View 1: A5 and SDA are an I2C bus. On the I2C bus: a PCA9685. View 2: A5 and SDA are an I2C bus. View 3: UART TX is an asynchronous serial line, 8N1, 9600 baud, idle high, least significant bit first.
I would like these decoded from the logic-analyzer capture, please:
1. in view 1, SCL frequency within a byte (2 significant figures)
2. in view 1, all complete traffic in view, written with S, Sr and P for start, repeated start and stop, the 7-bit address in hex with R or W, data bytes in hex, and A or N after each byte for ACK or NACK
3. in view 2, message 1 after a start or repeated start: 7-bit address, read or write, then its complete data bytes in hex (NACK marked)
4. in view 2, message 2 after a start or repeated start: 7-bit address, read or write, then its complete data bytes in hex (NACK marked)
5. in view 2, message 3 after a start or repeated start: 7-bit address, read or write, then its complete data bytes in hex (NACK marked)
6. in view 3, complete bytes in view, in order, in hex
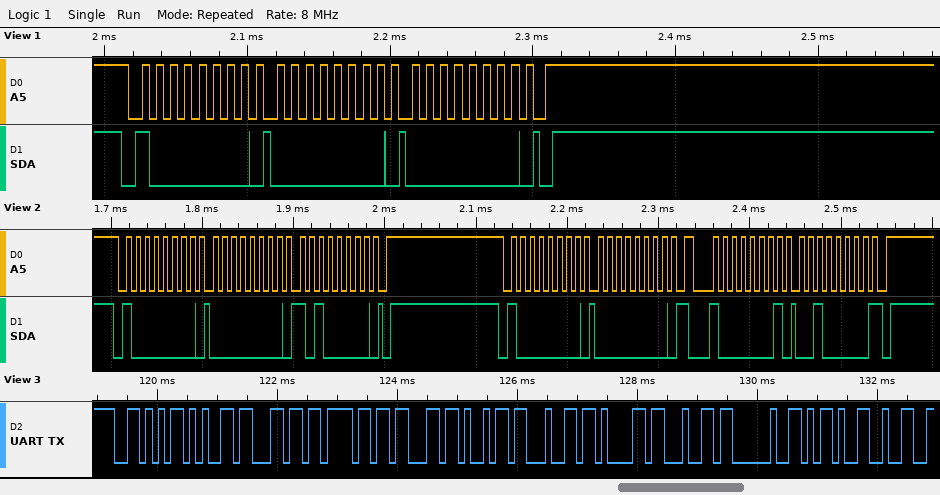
100 kHz
S 40W A 00 A 00 A P
0x40 write: 00 A0
0x40 write: 00
0x40 read: 20 NACK
56 65 6C 6F 63 69 64 61 64 20 2D 32
